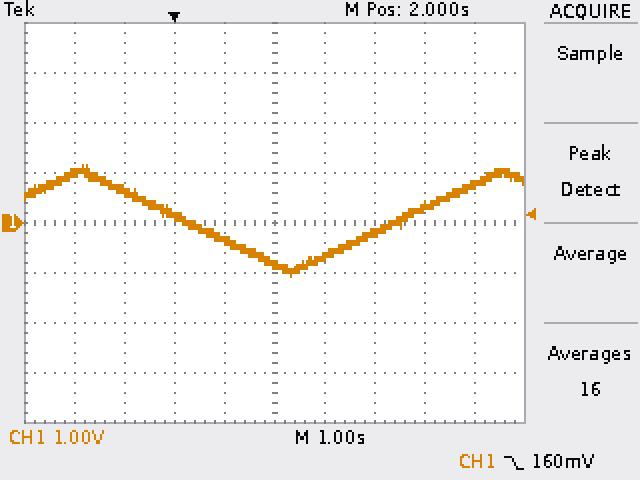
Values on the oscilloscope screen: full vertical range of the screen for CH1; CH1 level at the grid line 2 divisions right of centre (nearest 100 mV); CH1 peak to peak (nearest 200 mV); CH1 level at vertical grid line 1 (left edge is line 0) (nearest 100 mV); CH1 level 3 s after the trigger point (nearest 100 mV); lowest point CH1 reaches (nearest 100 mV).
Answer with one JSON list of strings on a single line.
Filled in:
["8 V", "-200 mV", "2.2 V", "1.0 V", "-700 mV", "-1.1 V"]
